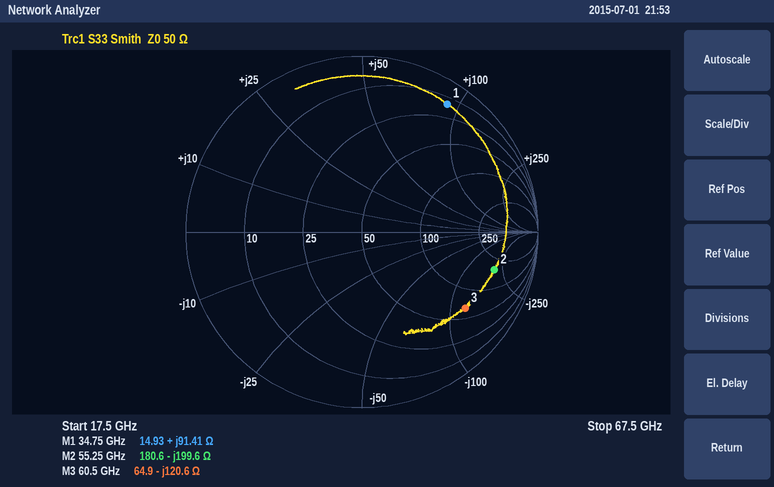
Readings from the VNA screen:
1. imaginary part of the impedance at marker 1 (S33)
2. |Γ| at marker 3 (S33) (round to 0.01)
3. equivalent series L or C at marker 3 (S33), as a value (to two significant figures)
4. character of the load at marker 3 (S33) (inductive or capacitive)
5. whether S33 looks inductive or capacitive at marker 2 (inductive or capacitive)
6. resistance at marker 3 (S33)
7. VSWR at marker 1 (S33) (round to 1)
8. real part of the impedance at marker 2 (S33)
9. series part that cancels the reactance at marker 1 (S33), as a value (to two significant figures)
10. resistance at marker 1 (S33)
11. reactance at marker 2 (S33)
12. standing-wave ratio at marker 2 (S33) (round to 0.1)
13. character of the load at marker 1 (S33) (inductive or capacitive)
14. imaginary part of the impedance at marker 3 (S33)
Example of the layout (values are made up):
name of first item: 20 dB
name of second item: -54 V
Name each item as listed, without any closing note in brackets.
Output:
imaginary part of the impedance at marker 1: +91.41 Ω
|Γ| at marker 3 (S33): 0.73
equivalent series L or C at marker 3 (S33), as a value: 22 fF
character of the load at marker 3 (S33): capacitive
whether S33 looks inductive or capacitive at marker 2: capacitive
resistance at marker 3: 64.9 Ω
VSWR at marker 1 (S33): 15
real part of the impedance at marker 2: 180.6 Ω
series part that cancels the reactance at marker 1 (S33), as a value: 50 fF
resistance at marker 1: 14.93 Ω
reactance at marker 2: -199.6 Ω
standing-wave ratio at marker 2 (S33): 8.2
character of the load at marker 1 (S33): inductive
imaginary part of the impedance at marker 3: -120.6 Ω
